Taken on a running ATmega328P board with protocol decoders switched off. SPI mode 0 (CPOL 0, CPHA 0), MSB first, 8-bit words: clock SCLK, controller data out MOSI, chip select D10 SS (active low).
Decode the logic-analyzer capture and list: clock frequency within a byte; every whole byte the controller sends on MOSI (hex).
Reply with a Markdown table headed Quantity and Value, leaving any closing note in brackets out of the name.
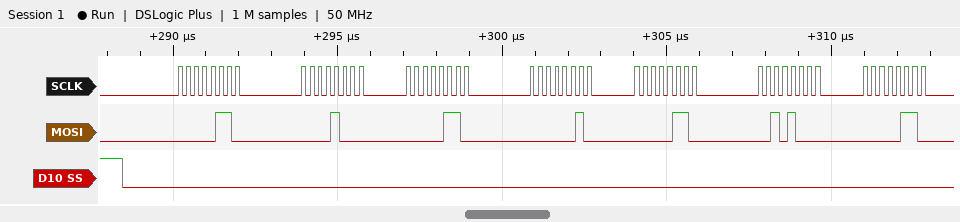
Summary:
| Quantity | Value |
|---|---|
| clock frequency within a byte | 4 MHz |
| every whole byte the controller sends on MOSI | 06 08 06 02 06 28 06 |
